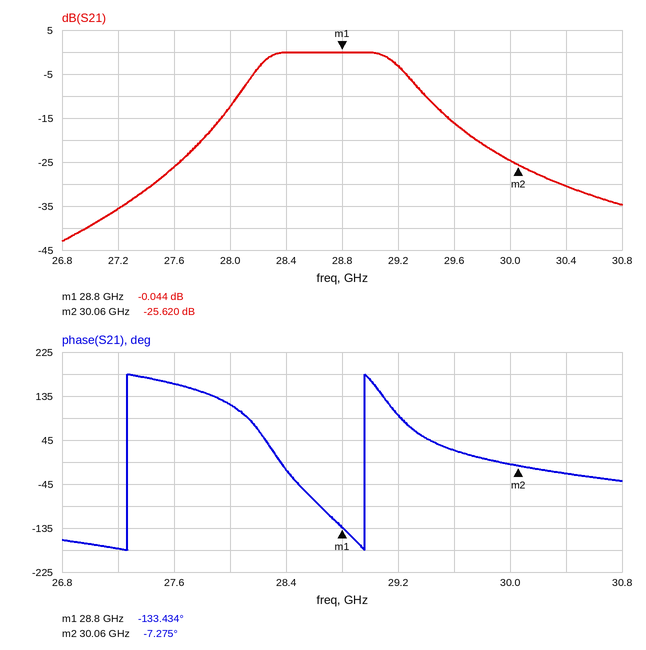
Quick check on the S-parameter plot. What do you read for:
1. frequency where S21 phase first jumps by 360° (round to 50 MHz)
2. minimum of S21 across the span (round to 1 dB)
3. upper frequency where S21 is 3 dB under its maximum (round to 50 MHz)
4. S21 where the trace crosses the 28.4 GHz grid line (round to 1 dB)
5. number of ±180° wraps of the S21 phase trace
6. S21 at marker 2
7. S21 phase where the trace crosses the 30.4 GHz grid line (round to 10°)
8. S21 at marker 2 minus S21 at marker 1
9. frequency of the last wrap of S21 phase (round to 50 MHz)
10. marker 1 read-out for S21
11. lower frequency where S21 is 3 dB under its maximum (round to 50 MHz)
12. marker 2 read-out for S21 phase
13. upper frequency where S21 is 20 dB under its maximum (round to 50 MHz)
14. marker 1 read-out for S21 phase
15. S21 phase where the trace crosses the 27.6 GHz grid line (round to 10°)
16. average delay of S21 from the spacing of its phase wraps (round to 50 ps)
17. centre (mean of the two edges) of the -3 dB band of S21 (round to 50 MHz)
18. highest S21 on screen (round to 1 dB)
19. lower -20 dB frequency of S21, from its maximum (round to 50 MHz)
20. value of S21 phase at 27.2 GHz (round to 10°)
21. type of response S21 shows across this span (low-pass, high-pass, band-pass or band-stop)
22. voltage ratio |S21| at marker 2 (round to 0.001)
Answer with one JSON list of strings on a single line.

["27.25 GHz", "-43 dB", "29.20 GHz", "0 dB", "2", "-25.620 dB", "-20°", "-25.576 dB", "28.95 GHz", "-0.044 dB", "28.20 GHz", "-7.275°", "29.75 GHz", "-133.434°", "160°", "600 ps", "28.70 GHz", "0 dB", "27.80 GHz", "-180°", "band-pass", "0.052"]
